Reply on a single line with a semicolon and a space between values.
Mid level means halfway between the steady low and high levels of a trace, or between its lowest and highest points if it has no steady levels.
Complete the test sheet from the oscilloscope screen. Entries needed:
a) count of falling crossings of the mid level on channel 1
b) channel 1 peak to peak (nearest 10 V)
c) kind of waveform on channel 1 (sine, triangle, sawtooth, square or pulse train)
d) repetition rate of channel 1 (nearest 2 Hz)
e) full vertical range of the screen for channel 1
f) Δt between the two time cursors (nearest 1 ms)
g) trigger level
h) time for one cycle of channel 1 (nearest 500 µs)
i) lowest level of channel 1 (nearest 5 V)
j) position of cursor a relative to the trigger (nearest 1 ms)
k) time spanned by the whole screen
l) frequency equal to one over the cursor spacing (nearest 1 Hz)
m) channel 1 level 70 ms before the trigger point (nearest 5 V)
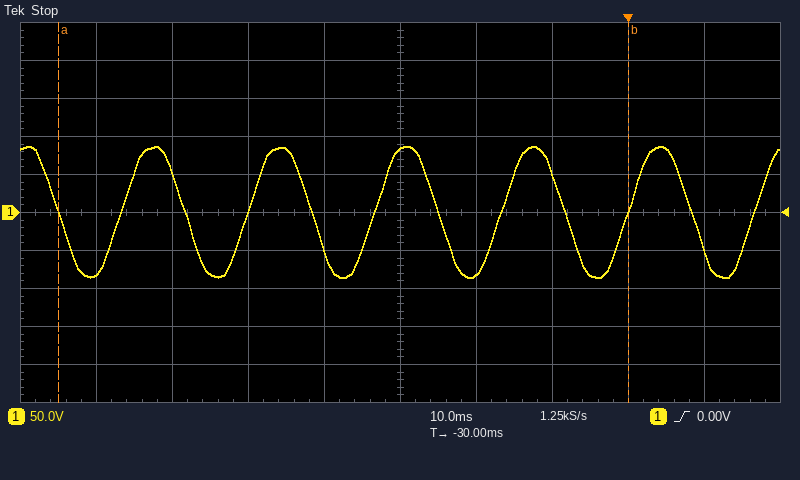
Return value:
6; 170 V; sine; 60 Hz; 500 V; 75 ms; 0.00 V; 16.5 ms; -85 V; -75 ms; 100 ms; 13 Hz; -80 V
